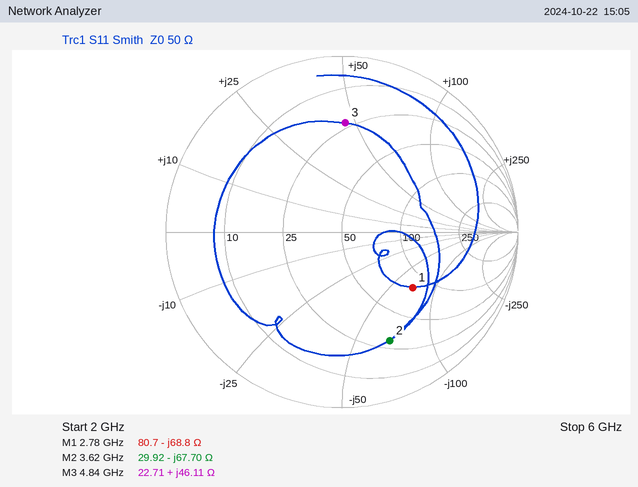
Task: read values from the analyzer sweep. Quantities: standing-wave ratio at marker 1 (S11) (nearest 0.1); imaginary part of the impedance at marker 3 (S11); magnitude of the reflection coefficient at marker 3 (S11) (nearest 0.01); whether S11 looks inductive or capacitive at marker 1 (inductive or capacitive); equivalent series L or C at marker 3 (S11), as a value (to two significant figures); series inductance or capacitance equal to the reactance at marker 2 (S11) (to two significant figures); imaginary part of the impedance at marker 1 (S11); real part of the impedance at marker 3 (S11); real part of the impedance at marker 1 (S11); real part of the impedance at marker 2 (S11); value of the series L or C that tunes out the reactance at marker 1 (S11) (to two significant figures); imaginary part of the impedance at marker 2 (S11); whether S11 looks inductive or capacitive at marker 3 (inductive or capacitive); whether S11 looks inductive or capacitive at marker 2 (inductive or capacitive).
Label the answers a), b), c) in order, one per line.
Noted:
a) 3.1
b) +46.11 Ω
c) 0.62
d) capacitive
e) 1.5 nH
f) 650 fF
g) -68.8 Ω
h) 22.71 Ω
i) 80.7 Ω
j) 29.92 Ω
k) 3.9 nH
l) -67.70 Ω
m) inductive
n) capacitive
